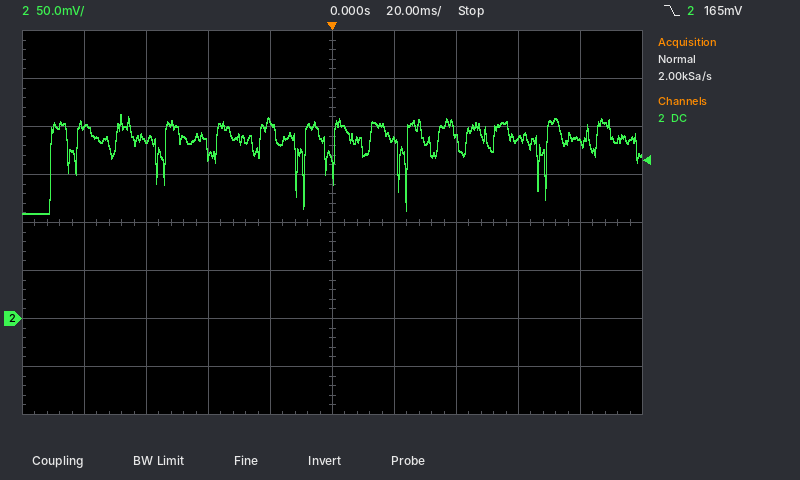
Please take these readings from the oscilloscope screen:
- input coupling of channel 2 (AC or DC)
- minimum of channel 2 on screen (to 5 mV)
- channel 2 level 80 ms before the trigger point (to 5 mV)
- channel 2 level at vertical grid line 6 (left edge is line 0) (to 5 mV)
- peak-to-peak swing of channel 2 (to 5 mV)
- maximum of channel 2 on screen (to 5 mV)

DC
110 mV
200 mV
185 mV
105 mV
215 mV
